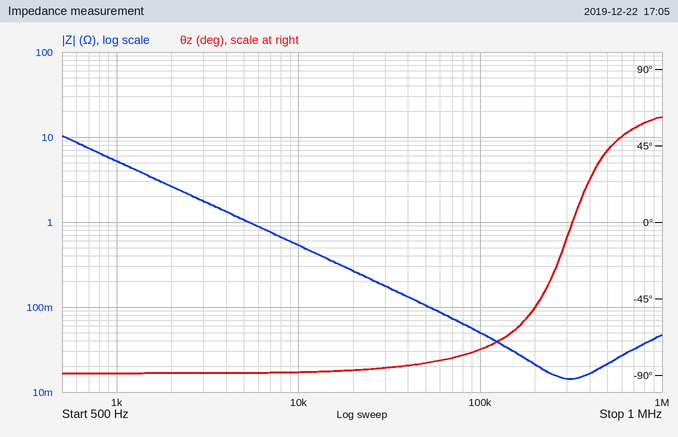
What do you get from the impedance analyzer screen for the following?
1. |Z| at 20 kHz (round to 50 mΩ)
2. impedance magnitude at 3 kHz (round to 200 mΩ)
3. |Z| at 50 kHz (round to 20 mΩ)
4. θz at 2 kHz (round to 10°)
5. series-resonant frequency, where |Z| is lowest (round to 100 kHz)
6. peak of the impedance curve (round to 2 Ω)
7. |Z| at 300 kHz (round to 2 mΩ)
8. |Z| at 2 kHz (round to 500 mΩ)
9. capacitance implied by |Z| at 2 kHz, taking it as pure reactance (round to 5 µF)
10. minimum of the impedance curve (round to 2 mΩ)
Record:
250 mΩ
1.8 Ω
100 mΩ
-90°
300 kHz
10 Ω
14 mΩ
2.5 Ω
30 µF
14 mΩ
